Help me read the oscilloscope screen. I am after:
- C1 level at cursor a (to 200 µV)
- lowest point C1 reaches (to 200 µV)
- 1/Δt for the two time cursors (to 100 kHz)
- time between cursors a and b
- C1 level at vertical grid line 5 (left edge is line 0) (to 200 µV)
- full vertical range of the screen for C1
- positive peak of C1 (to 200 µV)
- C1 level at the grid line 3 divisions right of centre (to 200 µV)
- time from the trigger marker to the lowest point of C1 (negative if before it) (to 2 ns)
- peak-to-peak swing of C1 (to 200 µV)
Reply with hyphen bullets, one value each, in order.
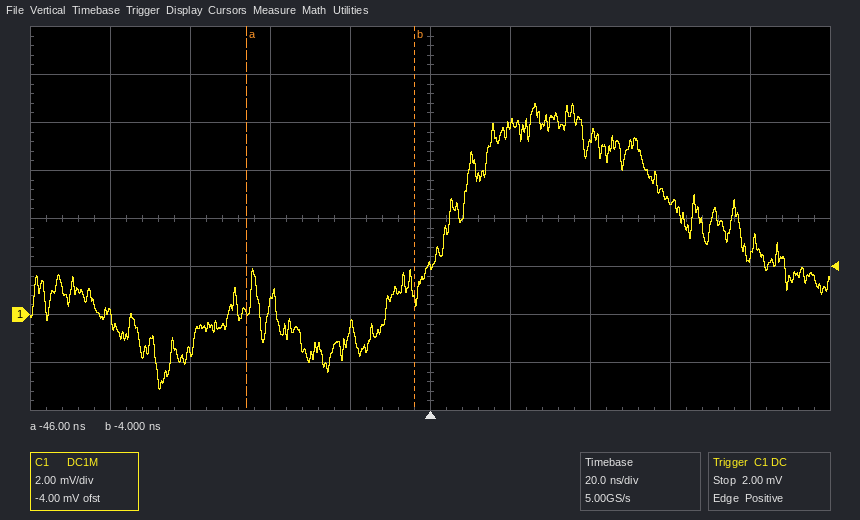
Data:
- 200 µV
- -3.2 mV
- 23.8 MHz
- 42 ns
- 2.0 mV
- 16 mV
- 8.8 mV
- 4.8 mV
- -68 ns
- 12.0 mV
